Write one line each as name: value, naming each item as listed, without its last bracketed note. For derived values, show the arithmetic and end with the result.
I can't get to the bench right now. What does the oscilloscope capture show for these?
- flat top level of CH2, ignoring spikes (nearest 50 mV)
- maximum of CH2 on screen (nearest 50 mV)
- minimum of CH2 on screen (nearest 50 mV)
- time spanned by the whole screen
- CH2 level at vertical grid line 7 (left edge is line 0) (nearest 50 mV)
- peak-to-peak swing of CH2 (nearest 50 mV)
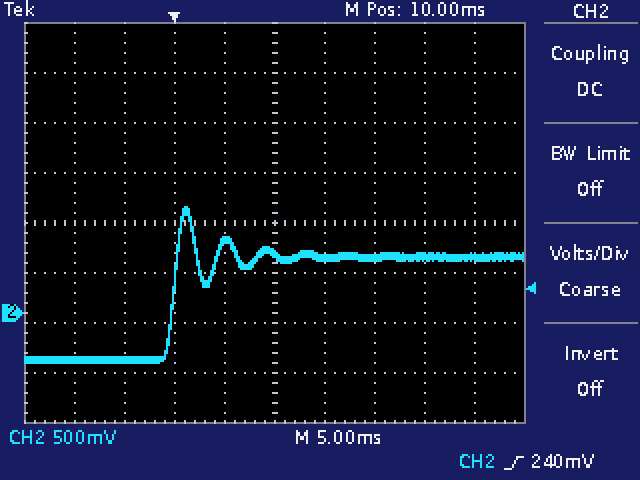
flat top level of CH2, ignoring spikes: 550 mV
maximum of CH2 on screen: 1.05 V
minimum of CH2 on screen: -500 mV
time spanned by the whole screen: 50 ms
CH2 level at vertical grid line 7 (left edge is line 0): 550 mV
peak-to-peak swing of CH2: 1.05 V − (-500 mV) = 1.55 V
